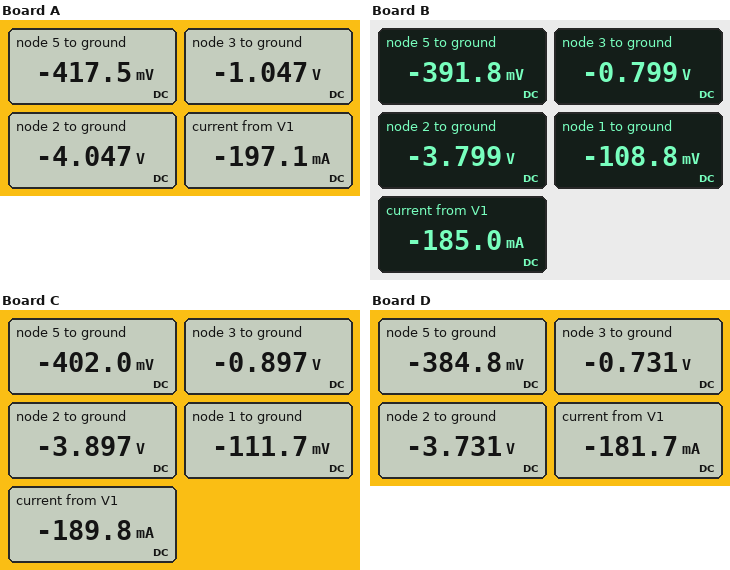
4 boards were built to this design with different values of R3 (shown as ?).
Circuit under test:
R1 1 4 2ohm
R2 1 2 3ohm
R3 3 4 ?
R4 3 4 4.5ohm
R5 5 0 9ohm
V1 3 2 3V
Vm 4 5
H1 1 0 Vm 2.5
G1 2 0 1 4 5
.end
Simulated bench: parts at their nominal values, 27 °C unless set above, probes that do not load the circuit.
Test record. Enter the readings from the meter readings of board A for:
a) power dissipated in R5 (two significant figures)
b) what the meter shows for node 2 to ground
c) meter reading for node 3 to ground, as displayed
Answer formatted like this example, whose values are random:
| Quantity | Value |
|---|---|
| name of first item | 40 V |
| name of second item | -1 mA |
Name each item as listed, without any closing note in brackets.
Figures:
| Quantity | Value |
|---|---|
| power dissipated in R5 | 19 mW |
| what the meter shows for node 2 to ground | -4.047 V |
| meter reading for node 3 to ground, as displayed | -1.047 V |
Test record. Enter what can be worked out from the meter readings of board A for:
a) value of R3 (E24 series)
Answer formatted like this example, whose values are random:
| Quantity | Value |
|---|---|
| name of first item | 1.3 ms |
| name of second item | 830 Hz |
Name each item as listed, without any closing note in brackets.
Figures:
| Quantity | Value |
|---|---|
| value of R3 | 11 Ω |
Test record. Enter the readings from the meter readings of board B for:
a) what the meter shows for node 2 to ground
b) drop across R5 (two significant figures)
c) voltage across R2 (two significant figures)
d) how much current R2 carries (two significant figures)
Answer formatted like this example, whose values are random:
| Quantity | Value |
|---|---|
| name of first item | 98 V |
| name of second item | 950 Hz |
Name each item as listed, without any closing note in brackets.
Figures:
| Quantity | Value |
|---|---|
| what the meter shows for node 2 to ground | -3.799 V |
| drop across R5 | 390 mV |
| voltage across R2 | 3.7 V |
| how much current R2 carries | 1.2 A |
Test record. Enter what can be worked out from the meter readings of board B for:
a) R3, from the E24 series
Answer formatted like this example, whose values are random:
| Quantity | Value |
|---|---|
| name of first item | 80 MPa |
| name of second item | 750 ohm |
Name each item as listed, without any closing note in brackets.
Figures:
| Quantity | Value |
|---|---|
| R3, from the E24 series | 4.3 Ω |
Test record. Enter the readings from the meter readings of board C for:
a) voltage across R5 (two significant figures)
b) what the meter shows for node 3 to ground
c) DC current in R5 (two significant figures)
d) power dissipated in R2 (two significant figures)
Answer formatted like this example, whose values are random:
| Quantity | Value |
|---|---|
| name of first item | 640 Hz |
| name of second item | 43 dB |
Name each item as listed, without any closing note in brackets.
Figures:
| Quantity | Value |
|---|---|
| voltage across R5 | 400 mV |
| what the meter shows for node 3 to ground | -0.897 V |
| DC current in R5 | 45 mA |
| power dissipated in R2 | 4.8 W |
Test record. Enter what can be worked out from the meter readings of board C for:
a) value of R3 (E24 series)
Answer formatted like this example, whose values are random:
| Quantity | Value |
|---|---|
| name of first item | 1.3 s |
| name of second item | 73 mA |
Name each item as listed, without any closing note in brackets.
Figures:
| Quantity | Value |
|---|---|
| value of R3 | 6.2 Ω |
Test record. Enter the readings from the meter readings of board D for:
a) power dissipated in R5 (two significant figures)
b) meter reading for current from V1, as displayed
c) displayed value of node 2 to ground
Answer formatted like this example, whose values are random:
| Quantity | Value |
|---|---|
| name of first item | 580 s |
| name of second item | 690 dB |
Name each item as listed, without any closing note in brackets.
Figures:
| Quantity | Value |
|---|---|
| power dissipated in R5 | 16 mW |
| meter reading for current from V1, as displayed | -181.7 mA |
| displayed value of node 2 to ground | -3.731 V |
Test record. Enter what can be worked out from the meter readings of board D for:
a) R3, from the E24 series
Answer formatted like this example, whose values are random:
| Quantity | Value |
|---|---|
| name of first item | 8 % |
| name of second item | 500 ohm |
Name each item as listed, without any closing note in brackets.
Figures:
| Quantity | Value |
|---|---|
| R3, from the E24 series | 3.3 Ω |
